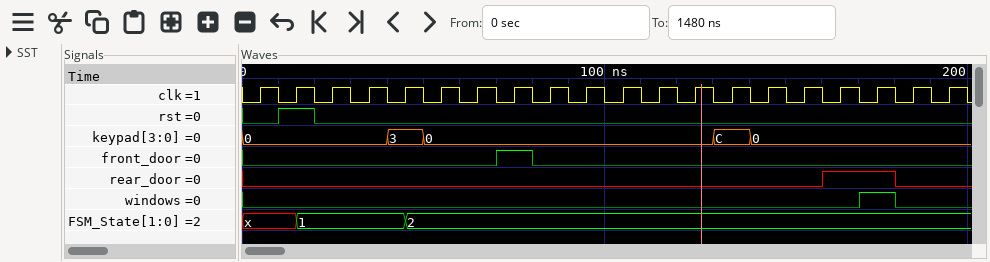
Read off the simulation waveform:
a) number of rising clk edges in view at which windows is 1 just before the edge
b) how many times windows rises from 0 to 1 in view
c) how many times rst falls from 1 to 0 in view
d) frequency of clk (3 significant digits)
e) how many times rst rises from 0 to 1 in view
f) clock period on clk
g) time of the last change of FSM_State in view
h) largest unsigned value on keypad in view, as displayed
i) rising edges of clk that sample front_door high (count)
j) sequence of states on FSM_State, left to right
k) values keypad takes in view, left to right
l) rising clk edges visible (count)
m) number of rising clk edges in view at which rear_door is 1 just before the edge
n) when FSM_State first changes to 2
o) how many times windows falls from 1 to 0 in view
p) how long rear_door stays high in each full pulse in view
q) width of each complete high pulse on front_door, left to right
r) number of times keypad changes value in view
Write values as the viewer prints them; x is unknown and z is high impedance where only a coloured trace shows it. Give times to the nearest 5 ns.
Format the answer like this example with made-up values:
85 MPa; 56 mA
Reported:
1; 1; 1; 100 MHz; 1; 10 ns; 45 ns; C; 1; x, 1, 2; 0, 3, 0, C, 0; 20; 2; 45 ns; 1; 20 ns; 10 ns; 4
